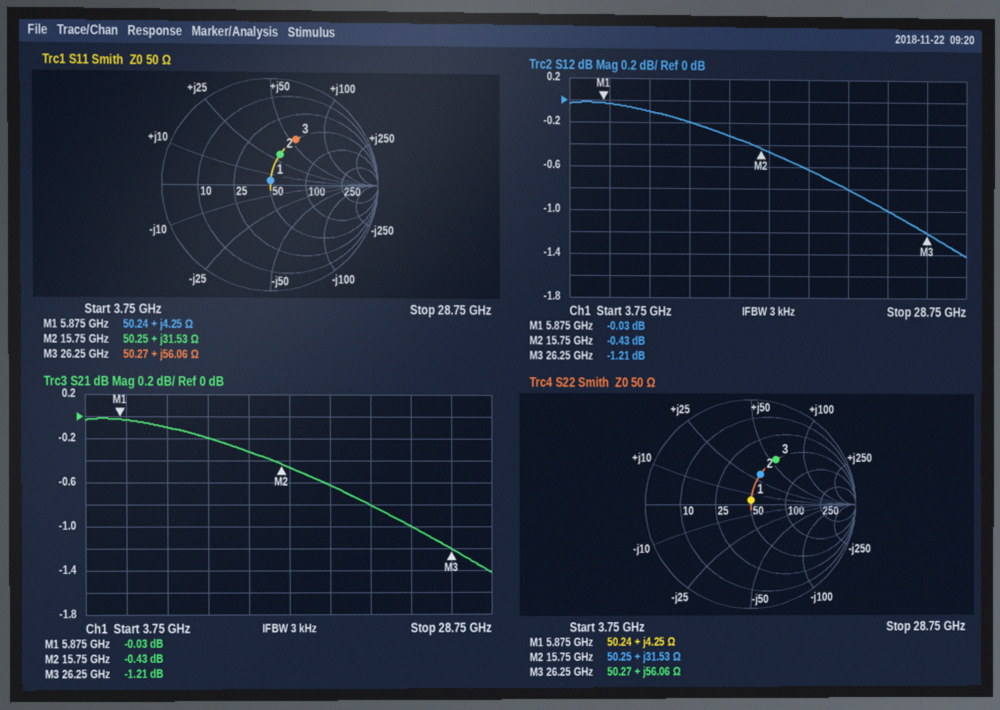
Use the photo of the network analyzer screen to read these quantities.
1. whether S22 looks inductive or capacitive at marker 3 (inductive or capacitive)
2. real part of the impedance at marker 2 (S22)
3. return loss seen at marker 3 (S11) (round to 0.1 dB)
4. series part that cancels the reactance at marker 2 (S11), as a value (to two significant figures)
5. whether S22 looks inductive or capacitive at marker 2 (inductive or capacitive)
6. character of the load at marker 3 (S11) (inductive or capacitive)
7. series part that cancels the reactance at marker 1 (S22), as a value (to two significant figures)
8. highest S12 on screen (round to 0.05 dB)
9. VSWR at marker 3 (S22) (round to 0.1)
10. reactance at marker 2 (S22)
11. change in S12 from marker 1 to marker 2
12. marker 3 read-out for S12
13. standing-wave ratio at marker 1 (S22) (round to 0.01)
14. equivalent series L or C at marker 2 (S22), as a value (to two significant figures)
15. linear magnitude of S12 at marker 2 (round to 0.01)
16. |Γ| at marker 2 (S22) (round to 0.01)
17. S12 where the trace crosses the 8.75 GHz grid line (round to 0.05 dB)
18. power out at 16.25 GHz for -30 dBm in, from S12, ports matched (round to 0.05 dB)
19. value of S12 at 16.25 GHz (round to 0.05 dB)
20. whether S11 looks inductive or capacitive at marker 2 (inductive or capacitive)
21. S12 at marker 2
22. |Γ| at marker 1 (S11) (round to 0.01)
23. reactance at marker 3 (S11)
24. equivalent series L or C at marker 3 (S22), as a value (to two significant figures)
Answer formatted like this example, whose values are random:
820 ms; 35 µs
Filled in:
inductive; 50.25 Ω; 6.2 dB; 320 fF; inductive; inductive; 6.4 pF; 0.00 dB; 2.9; +31.53 Ω; -0.40 dB; -1.21 dB; 1.09; 320 pH; 0.95; 0.30; -0.10 dB; -30.45 dBm; -0.45 dB; inductive; -0.43 dB; 0.04; +56.06 Ω; 340 pH
